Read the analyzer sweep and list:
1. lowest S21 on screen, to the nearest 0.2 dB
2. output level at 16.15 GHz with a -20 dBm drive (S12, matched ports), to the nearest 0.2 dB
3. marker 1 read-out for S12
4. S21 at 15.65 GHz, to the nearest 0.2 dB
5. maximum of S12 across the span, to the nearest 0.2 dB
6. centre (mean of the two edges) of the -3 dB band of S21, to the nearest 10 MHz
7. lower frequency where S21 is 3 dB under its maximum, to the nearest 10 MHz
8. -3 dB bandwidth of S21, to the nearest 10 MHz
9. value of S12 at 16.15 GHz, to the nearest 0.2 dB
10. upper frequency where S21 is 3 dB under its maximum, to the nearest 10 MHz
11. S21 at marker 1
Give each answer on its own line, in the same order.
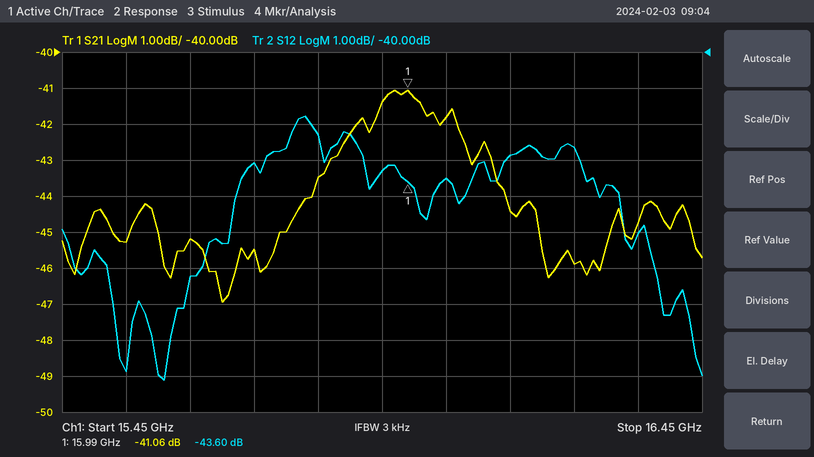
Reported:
-47.0 dB
-62.8 dBm
-43.60 dB
-45.2 dB
-41.8 dB
15.99 GHz
15.83 GHz
310 MHz
-42.8 dB
16.14 GHz
-41.06 dB
